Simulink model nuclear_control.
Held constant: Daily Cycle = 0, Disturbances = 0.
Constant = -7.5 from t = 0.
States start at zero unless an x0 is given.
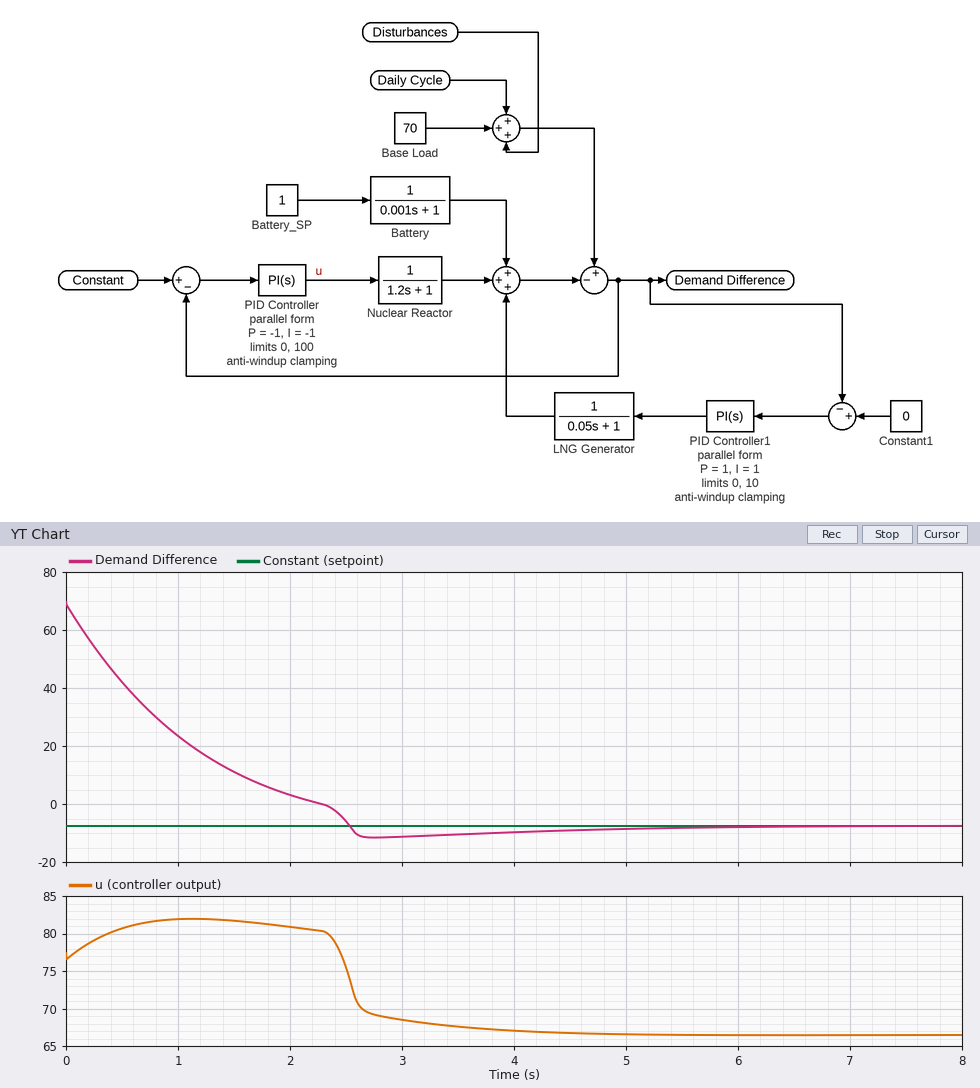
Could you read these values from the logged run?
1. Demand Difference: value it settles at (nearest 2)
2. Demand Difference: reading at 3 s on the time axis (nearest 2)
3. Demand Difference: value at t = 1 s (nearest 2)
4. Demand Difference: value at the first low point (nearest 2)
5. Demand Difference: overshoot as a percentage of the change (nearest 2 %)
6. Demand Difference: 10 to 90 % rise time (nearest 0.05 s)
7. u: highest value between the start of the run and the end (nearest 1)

-8
-12
24
-12
6 %
2.15 s
82
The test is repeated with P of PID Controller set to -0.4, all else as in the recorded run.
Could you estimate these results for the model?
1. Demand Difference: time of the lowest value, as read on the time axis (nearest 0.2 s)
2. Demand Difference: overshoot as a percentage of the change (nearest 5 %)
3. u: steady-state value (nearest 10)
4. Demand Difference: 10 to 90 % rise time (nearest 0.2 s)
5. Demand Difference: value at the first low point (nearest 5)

3.4 s
15 %
70
2.0 s
-20
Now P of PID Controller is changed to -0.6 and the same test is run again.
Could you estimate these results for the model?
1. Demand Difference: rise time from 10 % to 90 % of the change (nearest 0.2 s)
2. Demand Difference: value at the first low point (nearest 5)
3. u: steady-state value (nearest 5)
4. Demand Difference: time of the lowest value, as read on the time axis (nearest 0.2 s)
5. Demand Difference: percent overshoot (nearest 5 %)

2.0 s
-15
65
3.2 s
10 %
